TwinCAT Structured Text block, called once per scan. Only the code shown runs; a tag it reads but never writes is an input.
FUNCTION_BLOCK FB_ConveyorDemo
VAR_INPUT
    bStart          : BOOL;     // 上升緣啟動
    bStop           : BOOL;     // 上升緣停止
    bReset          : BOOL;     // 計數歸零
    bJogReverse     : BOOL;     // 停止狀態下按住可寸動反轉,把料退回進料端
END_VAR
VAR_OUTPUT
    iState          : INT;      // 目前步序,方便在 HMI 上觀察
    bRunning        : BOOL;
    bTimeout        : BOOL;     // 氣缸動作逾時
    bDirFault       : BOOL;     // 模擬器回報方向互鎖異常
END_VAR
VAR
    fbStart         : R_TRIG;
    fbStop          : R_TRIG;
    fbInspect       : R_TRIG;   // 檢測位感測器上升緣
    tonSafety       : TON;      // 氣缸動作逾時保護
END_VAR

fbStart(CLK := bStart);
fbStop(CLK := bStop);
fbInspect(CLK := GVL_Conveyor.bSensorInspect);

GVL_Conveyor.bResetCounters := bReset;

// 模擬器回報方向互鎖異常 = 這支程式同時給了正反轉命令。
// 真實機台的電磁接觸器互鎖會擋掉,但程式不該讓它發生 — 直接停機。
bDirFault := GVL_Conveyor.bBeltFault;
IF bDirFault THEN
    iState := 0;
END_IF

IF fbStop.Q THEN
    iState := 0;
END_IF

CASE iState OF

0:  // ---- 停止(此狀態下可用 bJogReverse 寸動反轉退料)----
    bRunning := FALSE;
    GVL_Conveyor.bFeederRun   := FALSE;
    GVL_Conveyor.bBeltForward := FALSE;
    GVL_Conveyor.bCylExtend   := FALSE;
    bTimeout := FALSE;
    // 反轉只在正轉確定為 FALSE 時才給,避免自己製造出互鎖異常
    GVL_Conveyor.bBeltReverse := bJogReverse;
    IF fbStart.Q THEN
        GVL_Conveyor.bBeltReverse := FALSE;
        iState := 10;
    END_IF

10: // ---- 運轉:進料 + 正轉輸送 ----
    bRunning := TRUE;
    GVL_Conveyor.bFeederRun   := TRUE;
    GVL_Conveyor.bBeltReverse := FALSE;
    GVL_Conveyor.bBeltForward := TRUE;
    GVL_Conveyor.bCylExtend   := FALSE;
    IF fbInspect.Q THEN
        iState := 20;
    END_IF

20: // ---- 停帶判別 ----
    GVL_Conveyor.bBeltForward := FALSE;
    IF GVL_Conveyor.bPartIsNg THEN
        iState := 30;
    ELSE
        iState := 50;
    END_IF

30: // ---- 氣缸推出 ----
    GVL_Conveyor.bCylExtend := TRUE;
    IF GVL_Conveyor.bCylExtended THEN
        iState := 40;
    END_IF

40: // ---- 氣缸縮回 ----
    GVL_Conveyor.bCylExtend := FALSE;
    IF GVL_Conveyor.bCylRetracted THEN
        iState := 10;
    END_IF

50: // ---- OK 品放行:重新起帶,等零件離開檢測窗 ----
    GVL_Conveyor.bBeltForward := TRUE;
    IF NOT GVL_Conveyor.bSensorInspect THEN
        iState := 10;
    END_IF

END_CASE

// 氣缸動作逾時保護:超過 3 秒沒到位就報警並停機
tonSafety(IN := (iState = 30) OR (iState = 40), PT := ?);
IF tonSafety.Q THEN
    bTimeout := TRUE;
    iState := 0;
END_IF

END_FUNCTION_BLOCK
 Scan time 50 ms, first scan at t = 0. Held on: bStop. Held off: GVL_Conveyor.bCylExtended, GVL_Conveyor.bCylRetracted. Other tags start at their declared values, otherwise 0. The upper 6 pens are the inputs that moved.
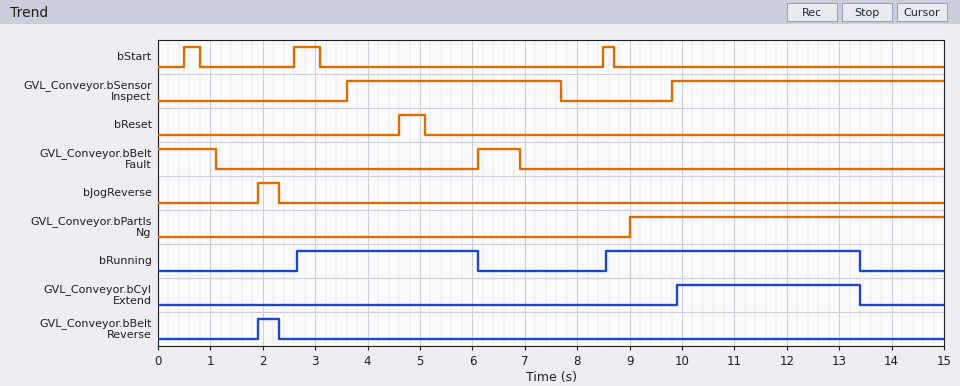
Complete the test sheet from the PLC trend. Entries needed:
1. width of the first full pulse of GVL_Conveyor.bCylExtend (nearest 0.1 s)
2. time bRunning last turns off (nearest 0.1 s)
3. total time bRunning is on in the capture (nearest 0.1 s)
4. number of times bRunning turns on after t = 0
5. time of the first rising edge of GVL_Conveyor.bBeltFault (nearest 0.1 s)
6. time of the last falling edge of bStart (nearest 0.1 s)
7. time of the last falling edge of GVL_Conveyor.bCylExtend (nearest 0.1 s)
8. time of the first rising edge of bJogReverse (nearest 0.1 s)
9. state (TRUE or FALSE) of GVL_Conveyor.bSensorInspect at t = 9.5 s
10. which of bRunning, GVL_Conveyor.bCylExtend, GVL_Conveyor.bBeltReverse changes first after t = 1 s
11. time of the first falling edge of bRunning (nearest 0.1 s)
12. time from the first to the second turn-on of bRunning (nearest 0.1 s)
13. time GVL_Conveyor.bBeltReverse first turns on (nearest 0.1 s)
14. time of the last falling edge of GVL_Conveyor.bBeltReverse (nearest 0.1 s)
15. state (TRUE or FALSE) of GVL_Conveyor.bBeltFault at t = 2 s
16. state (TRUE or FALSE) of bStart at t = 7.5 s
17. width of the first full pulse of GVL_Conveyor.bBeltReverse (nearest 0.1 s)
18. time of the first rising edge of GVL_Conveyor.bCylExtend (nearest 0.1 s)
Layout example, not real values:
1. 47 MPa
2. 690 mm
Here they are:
1. 3.5 s
2. 13.4 s
3. 8.3 s
4. 2
5. 6.1 s
6. 8.7 s
7. 13.4 s
8. 1.9 s
9. FALSE
10. GVL_Conveyor.bBeltReverse
11. 6.1 s
12. 5.9 s
13. 1.9 s
14. 2.3 s
15. FALSE
16. FALSE
17. 0.4 s
18. 9.9 s
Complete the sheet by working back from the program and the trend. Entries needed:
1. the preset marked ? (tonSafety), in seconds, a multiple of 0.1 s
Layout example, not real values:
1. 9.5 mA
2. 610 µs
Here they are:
1. 3.5 s
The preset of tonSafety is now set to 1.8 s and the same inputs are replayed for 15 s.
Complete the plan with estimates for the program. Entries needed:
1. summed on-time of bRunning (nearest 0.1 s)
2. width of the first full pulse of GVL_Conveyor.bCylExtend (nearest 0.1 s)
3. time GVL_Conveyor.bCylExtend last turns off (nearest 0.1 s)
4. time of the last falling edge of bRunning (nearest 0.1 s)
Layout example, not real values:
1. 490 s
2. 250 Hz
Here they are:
1. 6.6 s
2. 1.8 s
3. 11.7 s
4. 11.7 s
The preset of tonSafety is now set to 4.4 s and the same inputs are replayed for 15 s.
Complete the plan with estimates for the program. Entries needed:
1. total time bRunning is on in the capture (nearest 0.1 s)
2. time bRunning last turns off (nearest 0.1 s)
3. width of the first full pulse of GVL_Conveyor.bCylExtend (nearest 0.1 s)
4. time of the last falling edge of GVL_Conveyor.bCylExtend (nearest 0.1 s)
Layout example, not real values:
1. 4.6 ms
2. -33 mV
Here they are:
1. 9.2 s
2. 14.3 s
3. 4.4 s
4. 14.3 s
